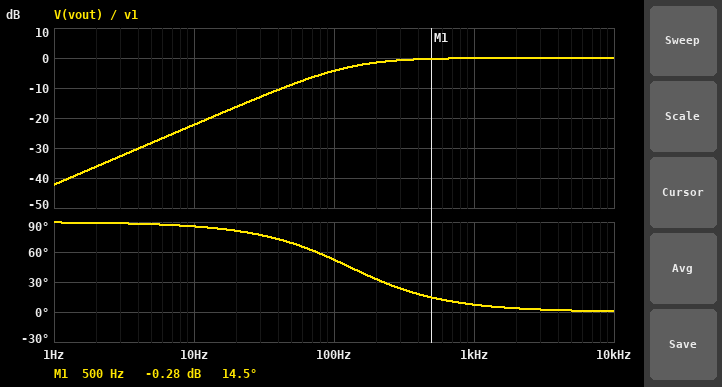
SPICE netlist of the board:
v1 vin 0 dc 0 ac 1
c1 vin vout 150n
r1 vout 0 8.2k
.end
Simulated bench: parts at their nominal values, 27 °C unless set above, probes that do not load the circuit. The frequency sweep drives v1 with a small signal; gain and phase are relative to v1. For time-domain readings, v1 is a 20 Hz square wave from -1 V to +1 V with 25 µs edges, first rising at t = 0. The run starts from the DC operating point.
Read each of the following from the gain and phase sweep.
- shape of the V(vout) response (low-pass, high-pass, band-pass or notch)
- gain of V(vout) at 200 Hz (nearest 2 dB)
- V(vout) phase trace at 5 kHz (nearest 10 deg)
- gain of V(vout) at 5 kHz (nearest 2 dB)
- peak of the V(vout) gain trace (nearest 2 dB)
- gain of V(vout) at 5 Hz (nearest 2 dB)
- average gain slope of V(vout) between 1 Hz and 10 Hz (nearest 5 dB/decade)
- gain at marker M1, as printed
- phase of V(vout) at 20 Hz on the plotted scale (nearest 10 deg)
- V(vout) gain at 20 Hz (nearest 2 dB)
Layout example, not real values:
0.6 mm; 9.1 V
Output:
high-pass; -2 dB; 0 deg; 0 dB; 0 dB; -28 dB; 20 dB/decade; -0.28 dB; 80 deg; -16 dB
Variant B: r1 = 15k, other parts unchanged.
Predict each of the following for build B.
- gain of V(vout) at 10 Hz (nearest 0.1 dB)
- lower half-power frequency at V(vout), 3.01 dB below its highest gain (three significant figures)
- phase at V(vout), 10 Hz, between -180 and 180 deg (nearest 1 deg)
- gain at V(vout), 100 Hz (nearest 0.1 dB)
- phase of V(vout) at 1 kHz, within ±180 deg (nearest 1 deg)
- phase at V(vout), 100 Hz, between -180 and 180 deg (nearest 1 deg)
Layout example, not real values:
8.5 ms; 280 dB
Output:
-17.1 dB; 70.7 Hz; 82 deg; -1.8 dB; 4 deg; 35 deg
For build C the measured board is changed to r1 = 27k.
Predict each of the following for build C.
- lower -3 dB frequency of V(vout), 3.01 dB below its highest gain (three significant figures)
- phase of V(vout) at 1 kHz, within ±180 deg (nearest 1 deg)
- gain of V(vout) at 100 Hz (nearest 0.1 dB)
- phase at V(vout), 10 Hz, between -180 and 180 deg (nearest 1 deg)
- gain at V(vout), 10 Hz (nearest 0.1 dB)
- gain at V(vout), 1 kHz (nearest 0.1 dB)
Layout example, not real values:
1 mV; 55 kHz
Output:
39.3 Hz; 2 deg; -0.6 dB; 76 deg; -12.2 dB; 0 dB
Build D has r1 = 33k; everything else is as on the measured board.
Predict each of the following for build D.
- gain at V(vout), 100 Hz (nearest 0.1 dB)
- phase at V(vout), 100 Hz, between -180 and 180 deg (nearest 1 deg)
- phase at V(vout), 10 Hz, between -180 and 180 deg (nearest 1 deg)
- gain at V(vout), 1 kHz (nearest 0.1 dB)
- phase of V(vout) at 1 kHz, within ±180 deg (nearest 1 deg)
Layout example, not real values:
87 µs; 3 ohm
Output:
-0.4 dB; 18 deg; 73 deg; 0 dB; 2 deg
